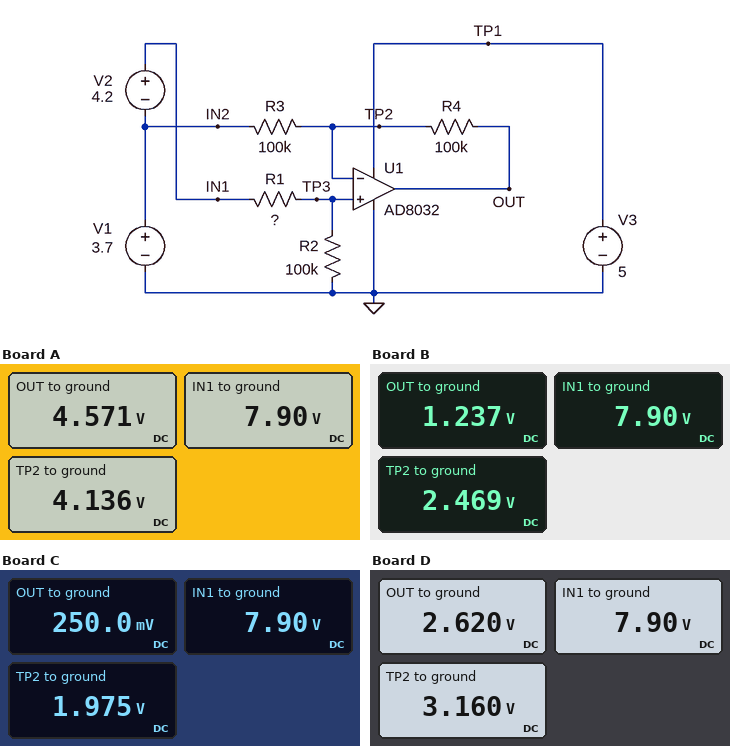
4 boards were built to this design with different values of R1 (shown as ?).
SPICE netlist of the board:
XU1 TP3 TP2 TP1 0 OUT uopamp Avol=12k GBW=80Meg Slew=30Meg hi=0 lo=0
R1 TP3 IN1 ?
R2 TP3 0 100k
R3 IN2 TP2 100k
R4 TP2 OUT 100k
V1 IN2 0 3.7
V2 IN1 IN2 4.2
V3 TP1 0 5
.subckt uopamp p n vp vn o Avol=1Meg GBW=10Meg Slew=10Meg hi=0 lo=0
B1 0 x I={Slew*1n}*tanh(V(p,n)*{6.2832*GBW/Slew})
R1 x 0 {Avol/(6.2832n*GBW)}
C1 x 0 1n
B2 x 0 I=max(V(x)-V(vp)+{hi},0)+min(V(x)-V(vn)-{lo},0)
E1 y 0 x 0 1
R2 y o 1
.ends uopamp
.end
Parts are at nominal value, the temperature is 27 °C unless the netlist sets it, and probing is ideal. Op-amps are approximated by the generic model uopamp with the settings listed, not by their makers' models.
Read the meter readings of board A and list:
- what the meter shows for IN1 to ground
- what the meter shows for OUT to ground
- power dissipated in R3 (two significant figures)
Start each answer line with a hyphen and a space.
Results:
- 7.90 V
- 4.571 V
- 1.9 µW
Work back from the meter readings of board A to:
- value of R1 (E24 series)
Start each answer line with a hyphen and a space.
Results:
- 91 kΩ
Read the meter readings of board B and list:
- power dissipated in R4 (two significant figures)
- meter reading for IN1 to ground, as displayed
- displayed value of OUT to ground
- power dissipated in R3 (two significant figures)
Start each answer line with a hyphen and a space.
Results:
- 15 µW
- 7.90 V
- 1.237 V
- 15 µW
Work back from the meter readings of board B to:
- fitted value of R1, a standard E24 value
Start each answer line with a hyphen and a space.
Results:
- 220 kΩ
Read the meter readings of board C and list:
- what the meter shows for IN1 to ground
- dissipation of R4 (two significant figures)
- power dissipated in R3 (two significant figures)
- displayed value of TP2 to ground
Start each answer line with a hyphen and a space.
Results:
- 7.90 V
- 30 µW
- 30 µW
- 1.975 V
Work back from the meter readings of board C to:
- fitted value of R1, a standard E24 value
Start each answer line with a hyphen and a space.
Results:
- 300 kΩ
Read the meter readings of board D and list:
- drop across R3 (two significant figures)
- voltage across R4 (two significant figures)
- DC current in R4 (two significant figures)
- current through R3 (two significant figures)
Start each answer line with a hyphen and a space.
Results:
- 540 mV
- 540 mV
- 5.4 µA
- 5.4 µA
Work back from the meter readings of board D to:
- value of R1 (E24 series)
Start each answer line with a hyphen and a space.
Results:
- 150 kΩ
